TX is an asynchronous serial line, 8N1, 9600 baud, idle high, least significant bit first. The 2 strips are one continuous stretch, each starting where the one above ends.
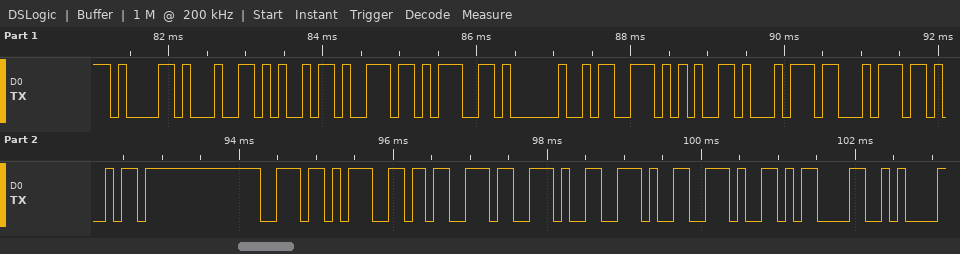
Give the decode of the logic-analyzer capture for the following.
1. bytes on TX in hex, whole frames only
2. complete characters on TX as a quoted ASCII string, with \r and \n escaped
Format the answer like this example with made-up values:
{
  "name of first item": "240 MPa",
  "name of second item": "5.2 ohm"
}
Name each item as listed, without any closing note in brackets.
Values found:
{
  "bytes on TX in hex, whole frames only": "61 64 69 6E 67 20 73 65 74 74 69 6E 67 73 2E 2E 2E 0D 0A",
  "complete characters on TX as a quoted ASCII string, with \\r and \\n escaped": "\"ading settings...\\r\\n\""
}
